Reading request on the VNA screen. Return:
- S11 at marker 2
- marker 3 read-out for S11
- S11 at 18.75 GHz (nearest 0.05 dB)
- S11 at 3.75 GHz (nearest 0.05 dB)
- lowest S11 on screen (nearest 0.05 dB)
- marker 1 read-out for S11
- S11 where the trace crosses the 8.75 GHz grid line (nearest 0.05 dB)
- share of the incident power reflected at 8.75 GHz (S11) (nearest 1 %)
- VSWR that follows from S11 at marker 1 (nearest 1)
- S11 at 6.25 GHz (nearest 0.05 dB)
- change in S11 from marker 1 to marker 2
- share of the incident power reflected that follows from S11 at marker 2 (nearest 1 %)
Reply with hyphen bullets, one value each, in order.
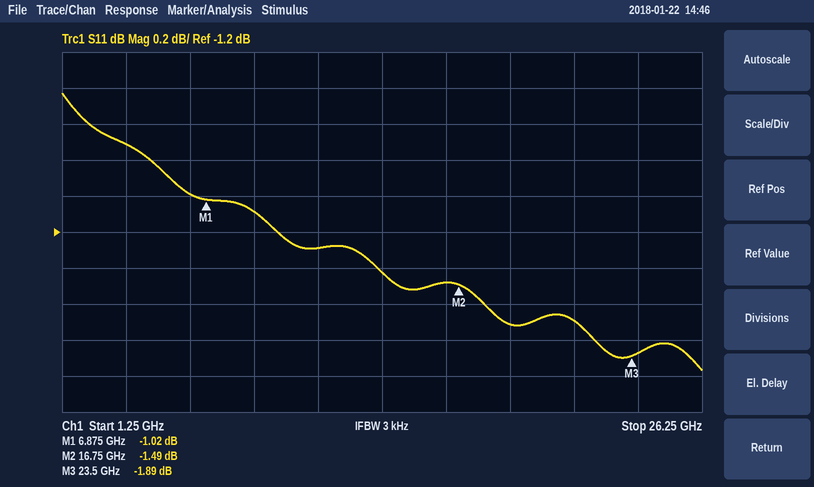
- -1.49 dB
- -1.89 dB
- -1.70 dB
- -0.70 dB
- -1.95 dB
- -1.02 dB
- -1.10 dB
- 78 %
- 17
- -1.00 dB
- -0.47 dB
- 71 %
